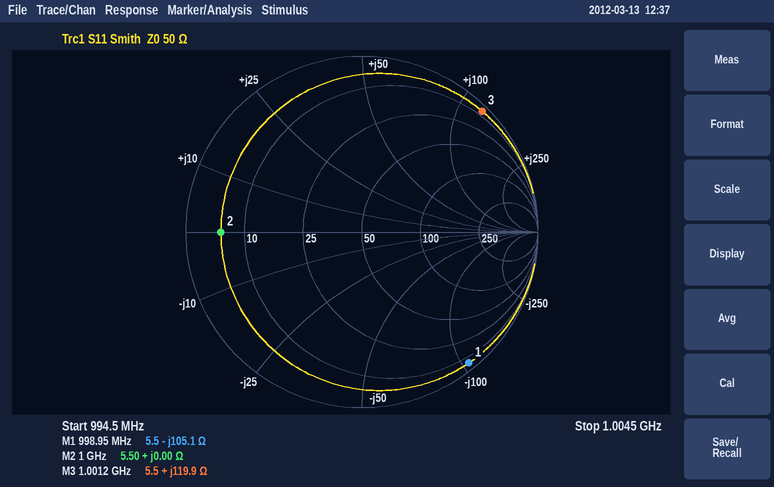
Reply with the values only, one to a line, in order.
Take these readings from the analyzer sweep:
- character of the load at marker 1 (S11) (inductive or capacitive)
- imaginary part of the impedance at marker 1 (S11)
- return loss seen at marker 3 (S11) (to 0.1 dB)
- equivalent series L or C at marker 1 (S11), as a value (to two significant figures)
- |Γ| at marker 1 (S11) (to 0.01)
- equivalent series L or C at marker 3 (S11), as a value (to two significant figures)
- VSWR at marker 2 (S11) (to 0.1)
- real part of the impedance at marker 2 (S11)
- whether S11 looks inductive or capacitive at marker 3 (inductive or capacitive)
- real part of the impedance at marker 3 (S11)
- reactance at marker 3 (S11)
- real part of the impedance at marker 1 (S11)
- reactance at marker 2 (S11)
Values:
capacitive
-105.1 Ω
0.3 dB
1.5 pF
0.96
19 nH
9.1
5.50 Ω
inductive
5.5 Ω
+119.9 Ω
5.5 Ω
+0.00 Ω
